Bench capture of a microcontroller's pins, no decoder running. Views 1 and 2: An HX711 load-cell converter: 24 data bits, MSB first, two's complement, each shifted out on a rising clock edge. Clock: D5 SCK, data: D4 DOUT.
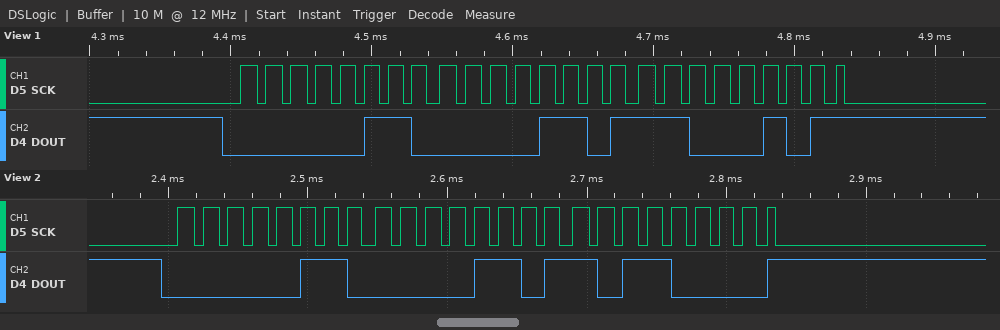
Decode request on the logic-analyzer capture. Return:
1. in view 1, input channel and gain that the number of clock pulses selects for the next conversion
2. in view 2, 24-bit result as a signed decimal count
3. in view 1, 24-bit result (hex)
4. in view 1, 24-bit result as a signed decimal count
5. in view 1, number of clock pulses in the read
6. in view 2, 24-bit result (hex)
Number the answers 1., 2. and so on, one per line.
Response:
1. channel A, gain 128
2. 396720
3. 0x060DC5
4. 396741
5. 25
6. 0x060DB0
